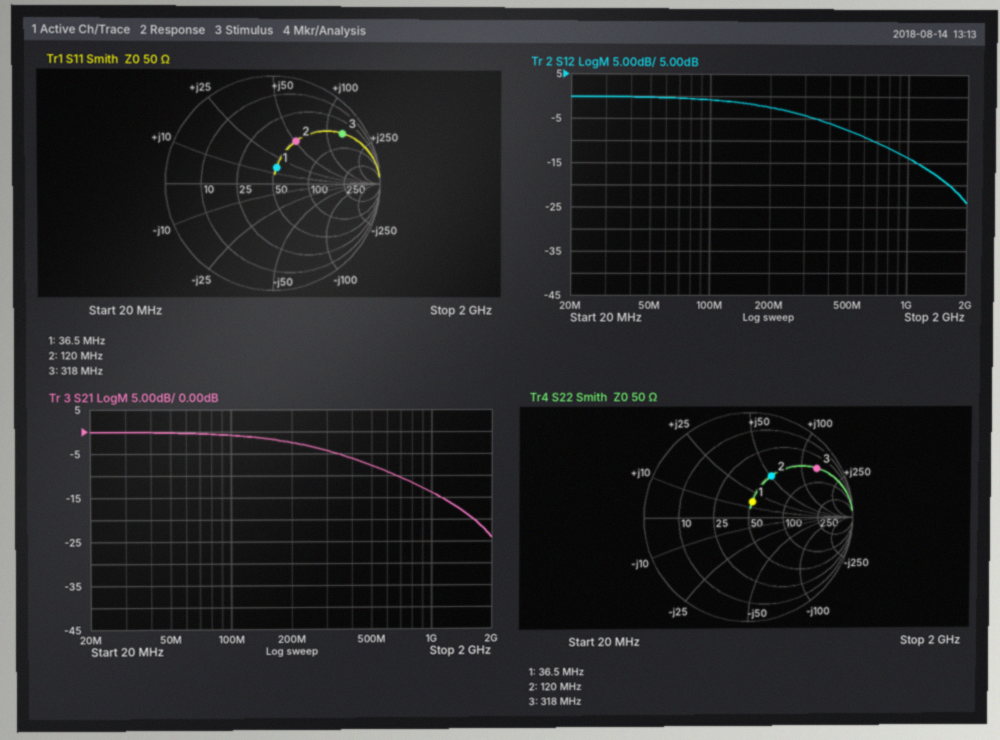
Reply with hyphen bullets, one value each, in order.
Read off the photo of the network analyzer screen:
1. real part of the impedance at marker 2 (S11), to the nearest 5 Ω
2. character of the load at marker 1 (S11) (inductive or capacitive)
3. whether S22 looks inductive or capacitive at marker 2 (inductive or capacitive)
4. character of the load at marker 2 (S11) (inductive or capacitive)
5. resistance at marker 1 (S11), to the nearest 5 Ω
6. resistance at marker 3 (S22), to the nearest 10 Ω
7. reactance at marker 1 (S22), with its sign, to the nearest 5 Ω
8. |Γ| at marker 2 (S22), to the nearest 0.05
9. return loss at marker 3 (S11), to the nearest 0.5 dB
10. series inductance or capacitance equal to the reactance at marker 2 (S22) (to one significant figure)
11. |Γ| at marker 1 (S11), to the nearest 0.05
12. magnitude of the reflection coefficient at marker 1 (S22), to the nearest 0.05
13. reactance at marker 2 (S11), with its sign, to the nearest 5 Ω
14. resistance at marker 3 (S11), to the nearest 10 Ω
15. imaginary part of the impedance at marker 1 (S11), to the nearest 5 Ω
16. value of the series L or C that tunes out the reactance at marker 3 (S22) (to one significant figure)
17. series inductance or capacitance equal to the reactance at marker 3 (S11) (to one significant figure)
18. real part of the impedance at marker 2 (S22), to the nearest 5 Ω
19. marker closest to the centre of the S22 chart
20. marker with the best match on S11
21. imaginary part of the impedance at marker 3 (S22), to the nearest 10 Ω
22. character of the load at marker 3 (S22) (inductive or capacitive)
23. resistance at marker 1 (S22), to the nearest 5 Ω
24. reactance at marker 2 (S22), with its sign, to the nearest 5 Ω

- 50 Ω
- inductive
- inductive
- inductive
- 50 Ω
- 50 Ω
- +15 Ω
- 0.45
- 2.0 dB
- 70 nH
- 0.15
- 0.15
- +50 Ω
- 50 Ω
- +15 Ω
- 4 pF
- 70 nH
- 50 Ω
- marker 1
- marker 1
- +140 Ω
- inductive
- 50 Ω
- +50 Ω
